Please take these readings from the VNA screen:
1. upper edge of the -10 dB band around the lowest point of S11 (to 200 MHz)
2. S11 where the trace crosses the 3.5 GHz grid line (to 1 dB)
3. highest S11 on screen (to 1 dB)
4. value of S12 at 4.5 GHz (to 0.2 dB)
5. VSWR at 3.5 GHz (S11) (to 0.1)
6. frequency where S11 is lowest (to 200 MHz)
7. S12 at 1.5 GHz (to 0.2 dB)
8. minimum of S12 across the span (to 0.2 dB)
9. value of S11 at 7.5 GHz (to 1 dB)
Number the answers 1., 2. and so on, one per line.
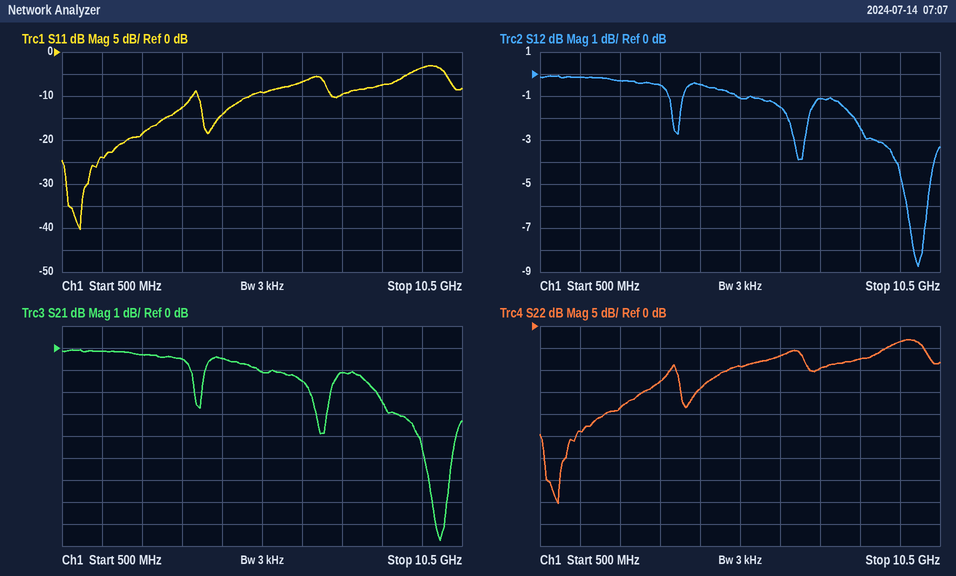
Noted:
1. 3.8 GHz
2. -13 dB
3. -3 dB
4. -0.4 dB
5. 1.6
6. 1.0 GHz
7. -0.2 dB
8. -8.8 dB
9. -10 dB
